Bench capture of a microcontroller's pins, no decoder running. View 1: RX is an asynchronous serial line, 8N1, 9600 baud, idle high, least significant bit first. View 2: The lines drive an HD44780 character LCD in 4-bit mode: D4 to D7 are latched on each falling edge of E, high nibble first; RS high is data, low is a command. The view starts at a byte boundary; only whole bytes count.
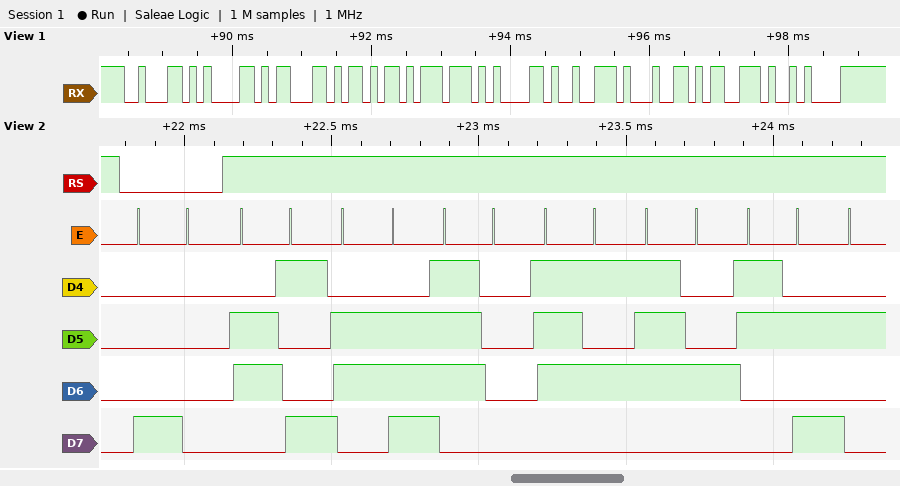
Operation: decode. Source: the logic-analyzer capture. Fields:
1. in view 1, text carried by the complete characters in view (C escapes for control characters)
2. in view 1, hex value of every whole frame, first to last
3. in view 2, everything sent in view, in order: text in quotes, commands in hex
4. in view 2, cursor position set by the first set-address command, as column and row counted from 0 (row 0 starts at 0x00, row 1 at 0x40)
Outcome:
"backwards\n"
0x62 0x61 0x63 0x6B 0x77 0x61 0x72 0x64 0x73 0x0A
0x80 "input:"
column 0, row 0
